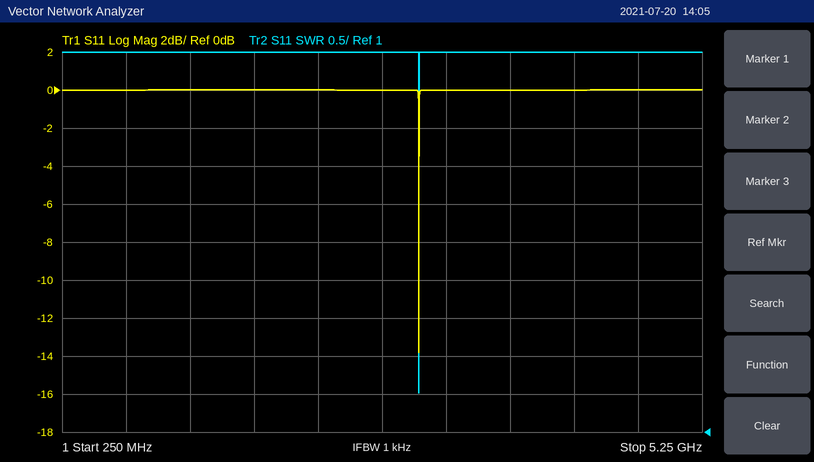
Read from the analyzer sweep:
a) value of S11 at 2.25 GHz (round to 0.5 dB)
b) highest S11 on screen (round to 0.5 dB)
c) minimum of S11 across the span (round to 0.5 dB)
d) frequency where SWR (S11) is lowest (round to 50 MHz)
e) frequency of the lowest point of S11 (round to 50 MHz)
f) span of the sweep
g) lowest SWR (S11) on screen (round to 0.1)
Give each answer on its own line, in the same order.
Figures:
0.0 dB
0.0 dB
-14.0 dB
3.05 GHz
3.05 GHz
5 GHz
1.5
